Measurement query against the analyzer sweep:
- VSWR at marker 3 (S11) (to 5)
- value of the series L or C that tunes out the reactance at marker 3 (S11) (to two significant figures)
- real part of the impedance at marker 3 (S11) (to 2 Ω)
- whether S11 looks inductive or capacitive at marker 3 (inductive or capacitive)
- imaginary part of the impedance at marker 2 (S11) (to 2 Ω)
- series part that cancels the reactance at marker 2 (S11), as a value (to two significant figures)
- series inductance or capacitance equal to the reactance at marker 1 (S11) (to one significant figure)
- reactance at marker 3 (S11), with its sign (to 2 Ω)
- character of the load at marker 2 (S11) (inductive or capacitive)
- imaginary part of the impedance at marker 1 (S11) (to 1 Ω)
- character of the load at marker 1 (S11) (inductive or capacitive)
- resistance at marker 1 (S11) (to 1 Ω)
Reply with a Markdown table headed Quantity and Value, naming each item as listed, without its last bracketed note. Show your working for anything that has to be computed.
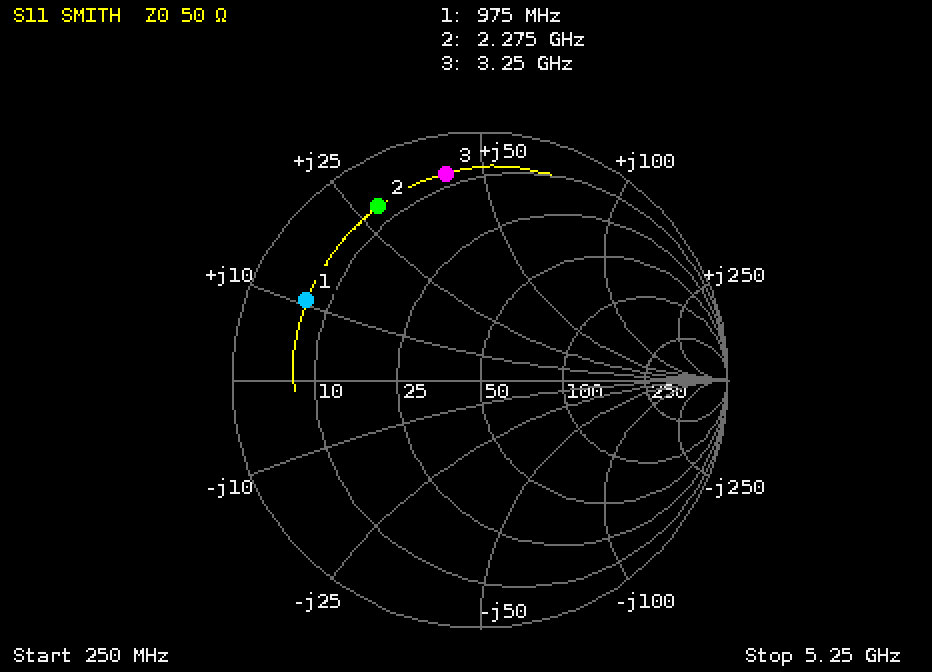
| Quantity | Value |
|---|---|
| VSWR at marker 3 (S11) | 10 |
| value of the series L or C that tunes out the reactance at marker 3 (S11) | C = 1/(2π × 3.25 GHz × 42 Ω) ≈ 1.2 pF |
| real part of the impedance at marker 3 (S11) | 8 Ω |
| whether S11 looks inductive or capacitive at marker 3 | inductive |
| imaginary part of the impedance at marker 2 (S11) | +28 Ω |
| series part that cancels the reactance at marker 2 (S11), as a value | C = 1/(2π × 2.275 GHz × 28 Ω) ≈ 2.5 pF |
| series inductance or capacitance equal to the reactance at marker 1 (S11) | L = 11 Ω/(2π × 975 MHz) ≈ 2 nH |
| reactance at marker 3 (S11), with its sign | +42 Ω |
| character of the load at marker 2 (S11) | inductive |
| imaginary part of the impedance at marker 1 (S11) | +11 Ω |
| character of the load at marker 1 (S11) | inductive |
| resistance at marker 1 (S11) | 7 Ω |
